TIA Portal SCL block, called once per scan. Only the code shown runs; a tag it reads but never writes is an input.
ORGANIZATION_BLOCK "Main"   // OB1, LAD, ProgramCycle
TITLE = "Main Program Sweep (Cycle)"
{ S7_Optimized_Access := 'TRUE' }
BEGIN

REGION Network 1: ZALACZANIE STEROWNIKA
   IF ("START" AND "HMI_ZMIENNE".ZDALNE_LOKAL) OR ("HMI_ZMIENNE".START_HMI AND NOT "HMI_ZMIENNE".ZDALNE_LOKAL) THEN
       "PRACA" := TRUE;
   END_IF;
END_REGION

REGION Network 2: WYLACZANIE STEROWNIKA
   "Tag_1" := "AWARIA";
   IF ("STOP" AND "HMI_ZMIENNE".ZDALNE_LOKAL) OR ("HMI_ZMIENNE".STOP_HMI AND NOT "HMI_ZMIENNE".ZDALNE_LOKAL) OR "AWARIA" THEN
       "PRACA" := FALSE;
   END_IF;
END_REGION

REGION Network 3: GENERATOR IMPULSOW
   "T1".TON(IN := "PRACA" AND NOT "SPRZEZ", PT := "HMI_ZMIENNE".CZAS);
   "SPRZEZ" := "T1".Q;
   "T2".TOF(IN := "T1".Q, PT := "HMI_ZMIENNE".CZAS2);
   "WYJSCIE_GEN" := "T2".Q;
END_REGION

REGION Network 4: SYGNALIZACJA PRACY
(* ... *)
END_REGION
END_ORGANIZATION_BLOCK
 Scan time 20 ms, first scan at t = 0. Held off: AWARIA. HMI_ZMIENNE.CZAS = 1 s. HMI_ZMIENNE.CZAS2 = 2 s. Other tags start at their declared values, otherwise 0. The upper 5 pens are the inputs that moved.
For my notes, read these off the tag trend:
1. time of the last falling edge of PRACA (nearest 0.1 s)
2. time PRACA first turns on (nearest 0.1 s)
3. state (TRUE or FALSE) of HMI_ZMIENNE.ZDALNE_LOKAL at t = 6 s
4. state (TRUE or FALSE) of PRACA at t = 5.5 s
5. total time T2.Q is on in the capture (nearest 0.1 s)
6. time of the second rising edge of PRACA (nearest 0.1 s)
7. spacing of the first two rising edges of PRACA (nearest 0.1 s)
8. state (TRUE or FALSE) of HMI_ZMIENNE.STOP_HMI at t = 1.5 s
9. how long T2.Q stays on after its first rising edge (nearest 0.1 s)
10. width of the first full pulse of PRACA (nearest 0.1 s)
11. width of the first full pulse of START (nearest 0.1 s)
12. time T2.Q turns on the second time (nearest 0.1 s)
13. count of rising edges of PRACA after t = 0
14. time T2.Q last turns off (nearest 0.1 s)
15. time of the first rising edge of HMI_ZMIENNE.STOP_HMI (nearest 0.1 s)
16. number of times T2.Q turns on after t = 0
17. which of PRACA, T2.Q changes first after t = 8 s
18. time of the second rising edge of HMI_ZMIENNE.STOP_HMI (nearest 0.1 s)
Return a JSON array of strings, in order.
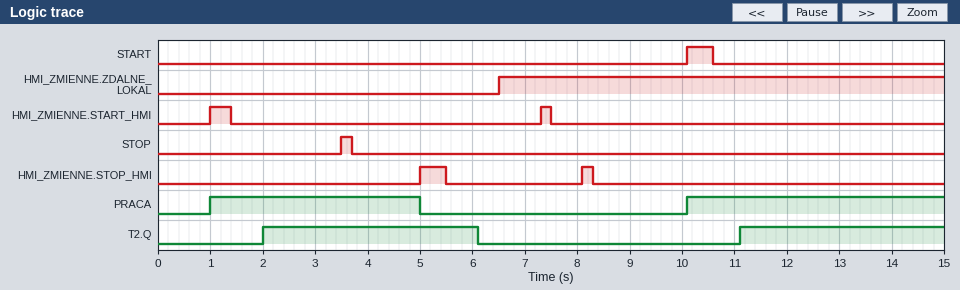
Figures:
["5.0 s", "1.0 s", "FALSE", "FALSE", "8.0 s", "10.1 s", "9.1 s", "FALSE", "4.1 s", "4.0 s", "0.5 s", "11.1 s", "2", "6.1 s", "5.0 s", "2", "PRACA", "8.1 s"]
